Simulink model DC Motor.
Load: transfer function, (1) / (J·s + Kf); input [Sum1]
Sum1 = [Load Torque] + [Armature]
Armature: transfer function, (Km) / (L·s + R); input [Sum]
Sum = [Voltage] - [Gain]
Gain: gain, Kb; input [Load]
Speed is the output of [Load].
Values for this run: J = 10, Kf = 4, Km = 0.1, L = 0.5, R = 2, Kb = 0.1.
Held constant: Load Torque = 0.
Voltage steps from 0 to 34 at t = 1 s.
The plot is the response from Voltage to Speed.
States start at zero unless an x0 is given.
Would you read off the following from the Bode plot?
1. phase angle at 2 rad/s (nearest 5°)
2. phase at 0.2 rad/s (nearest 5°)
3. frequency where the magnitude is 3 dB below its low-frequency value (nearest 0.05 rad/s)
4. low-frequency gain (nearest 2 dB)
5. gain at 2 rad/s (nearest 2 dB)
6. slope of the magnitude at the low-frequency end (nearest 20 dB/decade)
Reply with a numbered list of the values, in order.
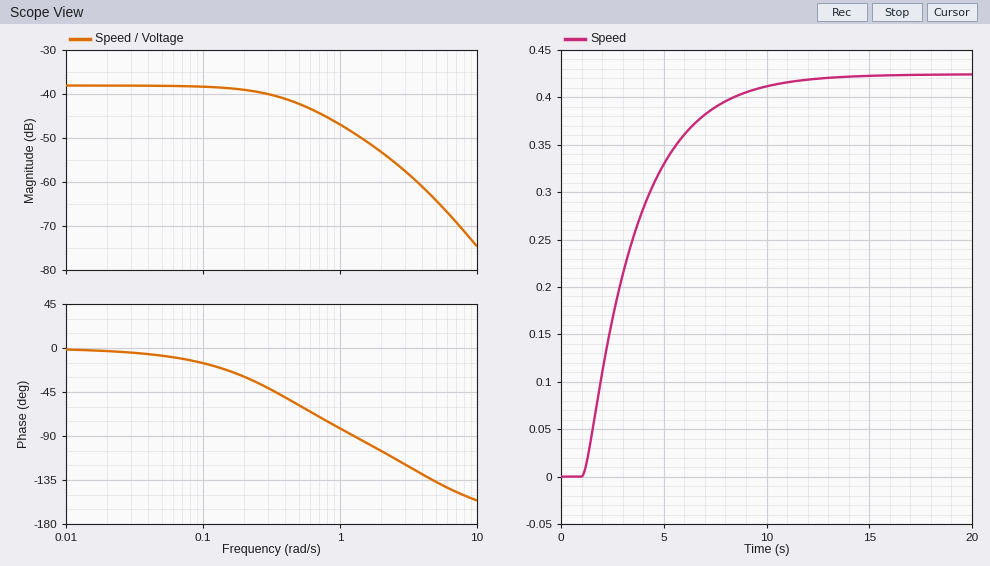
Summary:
1. -105°
2. -30°
3. 0.40 rad/s
4. -38 dB
5. -54 dB
6. 0 dB/decade
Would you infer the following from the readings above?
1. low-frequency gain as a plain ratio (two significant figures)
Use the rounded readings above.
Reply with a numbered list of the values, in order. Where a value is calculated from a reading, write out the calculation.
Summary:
1. 10^(-38 / 20) = 0.013
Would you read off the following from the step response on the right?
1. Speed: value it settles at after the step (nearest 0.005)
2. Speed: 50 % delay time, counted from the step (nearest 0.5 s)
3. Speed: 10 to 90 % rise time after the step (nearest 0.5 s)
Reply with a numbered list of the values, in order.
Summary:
1. 0.425
2. 2.0 s
3. 5.5 s
